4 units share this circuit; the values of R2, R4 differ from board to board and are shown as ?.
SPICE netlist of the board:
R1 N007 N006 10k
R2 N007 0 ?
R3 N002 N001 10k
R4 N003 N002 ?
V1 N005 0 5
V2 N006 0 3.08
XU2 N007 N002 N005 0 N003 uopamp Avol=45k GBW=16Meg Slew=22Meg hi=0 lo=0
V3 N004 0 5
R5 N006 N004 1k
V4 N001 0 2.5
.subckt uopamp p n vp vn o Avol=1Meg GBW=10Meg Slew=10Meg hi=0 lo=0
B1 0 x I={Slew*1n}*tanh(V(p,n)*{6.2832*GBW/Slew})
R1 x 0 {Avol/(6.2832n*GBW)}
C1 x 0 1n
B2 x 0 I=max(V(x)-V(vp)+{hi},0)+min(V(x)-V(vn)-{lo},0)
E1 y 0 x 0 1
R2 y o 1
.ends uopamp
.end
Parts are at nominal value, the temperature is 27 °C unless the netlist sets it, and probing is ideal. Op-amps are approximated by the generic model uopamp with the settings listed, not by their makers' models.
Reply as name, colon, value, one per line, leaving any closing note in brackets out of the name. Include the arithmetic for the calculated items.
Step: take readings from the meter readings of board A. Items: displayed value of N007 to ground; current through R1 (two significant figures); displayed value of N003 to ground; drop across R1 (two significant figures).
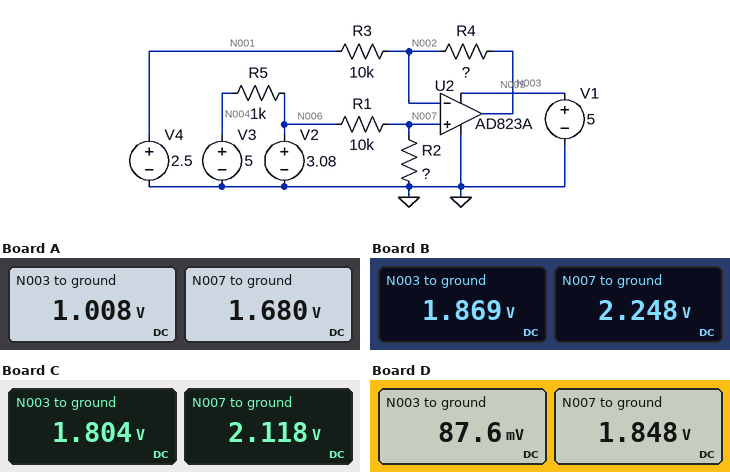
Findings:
displayed value of N007 to ground: 1.680 V
current through R1: (3.08 V - 1.68 V) / 10 kΩ = 140 µA
displayed value of N003 to ground: 1.008 V
drop across R1: 3.08 V - 1.68 V = 1.4 V
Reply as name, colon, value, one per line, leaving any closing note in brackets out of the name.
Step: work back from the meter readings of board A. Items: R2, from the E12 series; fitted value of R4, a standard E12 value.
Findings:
R2, from the E12 series: 12 kΩ
fitted value of R4, a standard E12 value: 8.2 kΩ
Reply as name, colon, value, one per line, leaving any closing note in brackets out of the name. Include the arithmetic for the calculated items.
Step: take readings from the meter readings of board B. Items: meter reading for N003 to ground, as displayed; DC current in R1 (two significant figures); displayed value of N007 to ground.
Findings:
meter reading for N003 to ground, as displayed: 1.869 V
DC current in R1: (3.08 V - 2.248 V) / 10 kΩ = 83 µA
displayed value of N007 to ground: 2.248 V
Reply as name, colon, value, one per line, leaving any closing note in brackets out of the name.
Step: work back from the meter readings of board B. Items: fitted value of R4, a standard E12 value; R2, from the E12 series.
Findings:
fitted value of R4, a standard E12 value: 15 kΩ
R2, from the E12 series: 27 kΩ
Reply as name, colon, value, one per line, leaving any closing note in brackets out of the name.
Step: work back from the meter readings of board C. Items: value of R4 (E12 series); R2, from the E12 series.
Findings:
value of R4: 8.2 kΩ
R2, from the E12 series: 22 kΩ
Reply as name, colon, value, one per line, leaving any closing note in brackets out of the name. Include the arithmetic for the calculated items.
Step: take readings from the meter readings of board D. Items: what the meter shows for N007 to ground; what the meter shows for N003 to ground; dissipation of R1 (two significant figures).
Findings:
what the meter shows for N007 to ground: 1.848 V
what the meter shows for N003 to ground: 87.6 mV
dissipation of R1: (3.08 V - 1.848 V)^2 / 10 kΩ = 150 µW
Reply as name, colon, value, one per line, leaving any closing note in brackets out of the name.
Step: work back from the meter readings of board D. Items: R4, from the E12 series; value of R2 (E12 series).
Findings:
R4, from the E12 series: 27 kΩ
value of R2: 15 kΩ
